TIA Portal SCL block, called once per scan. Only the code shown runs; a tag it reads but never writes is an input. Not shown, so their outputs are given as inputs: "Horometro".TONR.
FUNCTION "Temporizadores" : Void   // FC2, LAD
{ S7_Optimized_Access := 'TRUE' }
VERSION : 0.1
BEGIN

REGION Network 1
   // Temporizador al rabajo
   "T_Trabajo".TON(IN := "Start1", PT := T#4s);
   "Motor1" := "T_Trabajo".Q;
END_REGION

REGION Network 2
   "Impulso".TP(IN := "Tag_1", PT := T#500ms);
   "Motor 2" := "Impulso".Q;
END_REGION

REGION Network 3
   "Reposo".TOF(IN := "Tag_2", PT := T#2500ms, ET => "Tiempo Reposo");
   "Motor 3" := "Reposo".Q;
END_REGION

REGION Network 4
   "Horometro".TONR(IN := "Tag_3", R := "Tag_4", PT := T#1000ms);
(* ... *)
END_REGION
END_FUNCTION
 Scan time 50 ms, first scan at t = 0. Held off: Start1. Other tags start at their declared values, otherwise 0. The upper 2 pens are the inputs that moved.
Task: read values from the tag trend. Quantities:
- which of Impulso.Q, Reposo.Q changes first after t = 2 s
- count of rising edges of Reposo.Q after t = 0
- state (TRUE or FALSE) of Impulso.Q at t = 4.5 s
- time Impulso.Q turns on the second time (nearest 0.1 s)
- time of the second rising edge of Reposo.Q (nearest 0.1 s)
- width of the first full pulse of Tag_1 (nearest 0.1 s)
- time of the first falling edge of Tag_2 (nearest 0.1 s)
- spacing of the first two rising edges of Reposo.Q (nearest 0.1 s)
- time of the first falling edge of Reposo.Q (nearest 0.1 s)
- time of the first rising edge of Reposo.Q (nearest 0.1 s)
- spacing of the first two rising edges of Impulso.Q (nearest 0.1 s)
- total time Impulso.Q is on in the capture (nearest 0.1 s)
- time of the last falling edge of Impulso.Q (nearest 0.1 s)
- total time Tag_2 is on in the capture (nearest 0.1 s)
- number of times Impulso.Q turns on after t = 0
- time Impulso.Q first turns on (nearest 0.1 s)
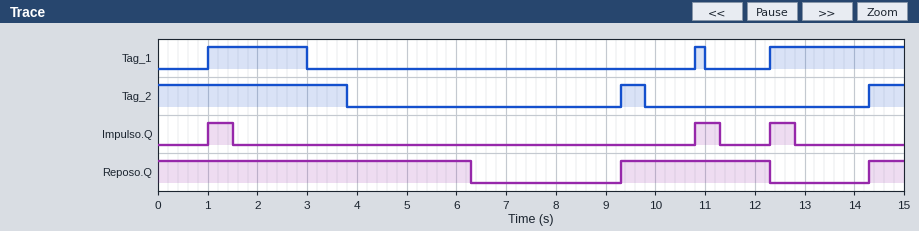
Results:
Reposo.Q
2
FALSE
10.8 s
14.3 s
2.0 s
3.8 s
5.0 s
6.3 s
9.3 s
9.8 s
1.5 s
12.8 s
5.0 s
3
1.0 s
